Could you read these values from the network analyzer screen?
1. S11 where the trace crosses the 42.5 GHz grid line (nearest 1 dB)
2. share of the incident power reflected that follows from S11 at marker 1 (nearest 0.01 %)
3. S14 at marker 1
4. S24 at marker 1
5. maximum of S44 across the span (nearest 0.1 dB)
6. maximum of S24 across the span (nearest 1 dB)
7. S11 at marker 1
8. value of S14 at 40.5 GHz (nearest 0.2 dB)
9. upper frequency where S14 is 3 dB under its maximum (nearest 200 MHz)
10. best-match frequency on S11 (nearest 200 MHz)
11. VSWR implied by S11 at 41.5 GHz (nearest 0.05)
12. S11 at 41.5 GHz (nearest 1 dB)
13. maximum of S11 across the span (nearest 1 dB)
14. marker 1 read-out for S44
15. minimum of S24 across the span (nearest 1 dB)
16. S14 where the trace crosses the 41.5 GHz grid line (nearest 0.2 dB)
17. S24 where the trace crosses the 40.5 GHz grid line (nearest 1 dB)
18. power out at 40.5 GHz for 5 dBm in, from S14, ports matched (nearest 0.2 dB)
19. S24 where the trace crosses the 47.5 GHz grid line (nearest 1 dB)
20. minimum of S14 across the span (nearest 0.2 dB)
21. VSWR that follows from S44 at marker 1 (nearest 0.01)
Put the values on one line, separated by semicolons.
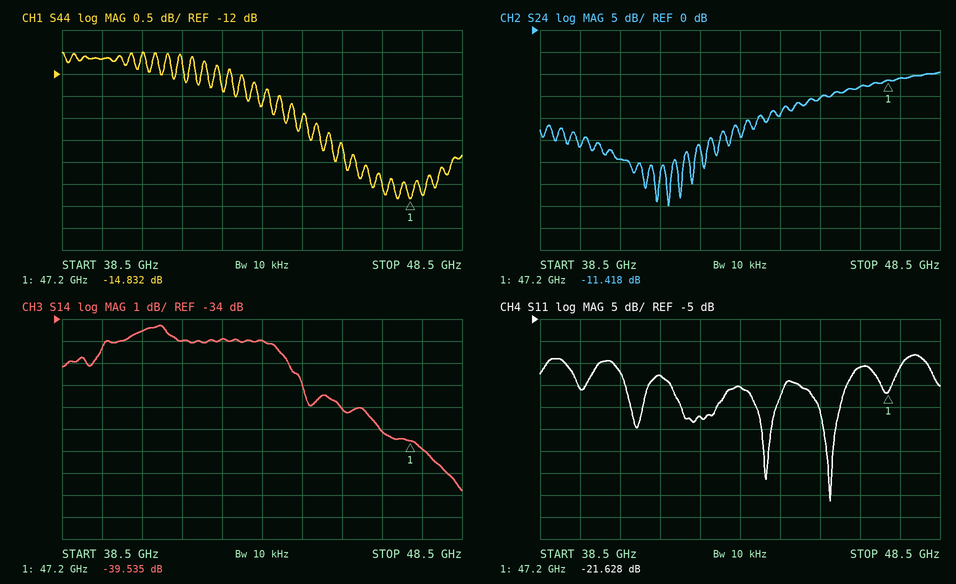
-27 dB; 0.69 %; -39.535 dB; -11.418 dB; -11.5 dB; -10 dB; -21.628 dB; -34.6 dB; 44.6 GHz; 45.8 GHz; 1.30; -18 dB; -13 dB; -14.832 dB; -40 dB; -35.0 dB; -29 dB; -29.6 dBm; -11 dB; -41.8 dB; 1.44
